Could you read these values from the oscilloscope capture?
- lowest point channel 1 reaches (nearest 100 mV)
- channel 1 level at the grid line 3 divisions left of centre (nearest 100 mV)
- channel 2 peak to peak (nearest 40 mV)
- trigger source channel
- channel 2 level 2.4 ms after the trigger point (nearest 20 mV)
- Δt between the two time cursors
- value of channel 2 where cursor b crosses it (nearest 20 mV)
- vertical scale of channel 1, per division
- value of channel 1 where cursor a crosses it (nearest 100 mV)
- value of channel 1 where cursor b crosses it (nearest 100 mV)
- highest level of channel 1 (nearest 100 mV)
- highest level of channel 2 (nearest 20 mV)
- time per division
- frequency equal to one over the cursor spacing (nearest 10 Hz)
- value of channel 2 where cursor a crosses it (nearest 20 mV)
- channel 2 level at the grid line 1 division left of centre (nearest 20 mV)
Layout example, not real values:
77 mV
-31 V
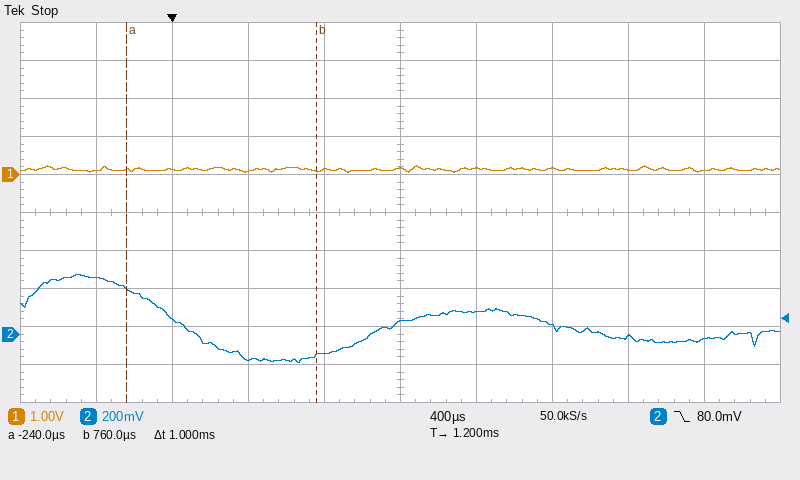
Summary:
100 mV
100 mV
480 mV
channel 2
-20 mV
1 ms
-120 mV
1 V
100 mV
100 mV
200 mV
320 mV
400 µs
1.00 kHz
240 mV
-100 mV
